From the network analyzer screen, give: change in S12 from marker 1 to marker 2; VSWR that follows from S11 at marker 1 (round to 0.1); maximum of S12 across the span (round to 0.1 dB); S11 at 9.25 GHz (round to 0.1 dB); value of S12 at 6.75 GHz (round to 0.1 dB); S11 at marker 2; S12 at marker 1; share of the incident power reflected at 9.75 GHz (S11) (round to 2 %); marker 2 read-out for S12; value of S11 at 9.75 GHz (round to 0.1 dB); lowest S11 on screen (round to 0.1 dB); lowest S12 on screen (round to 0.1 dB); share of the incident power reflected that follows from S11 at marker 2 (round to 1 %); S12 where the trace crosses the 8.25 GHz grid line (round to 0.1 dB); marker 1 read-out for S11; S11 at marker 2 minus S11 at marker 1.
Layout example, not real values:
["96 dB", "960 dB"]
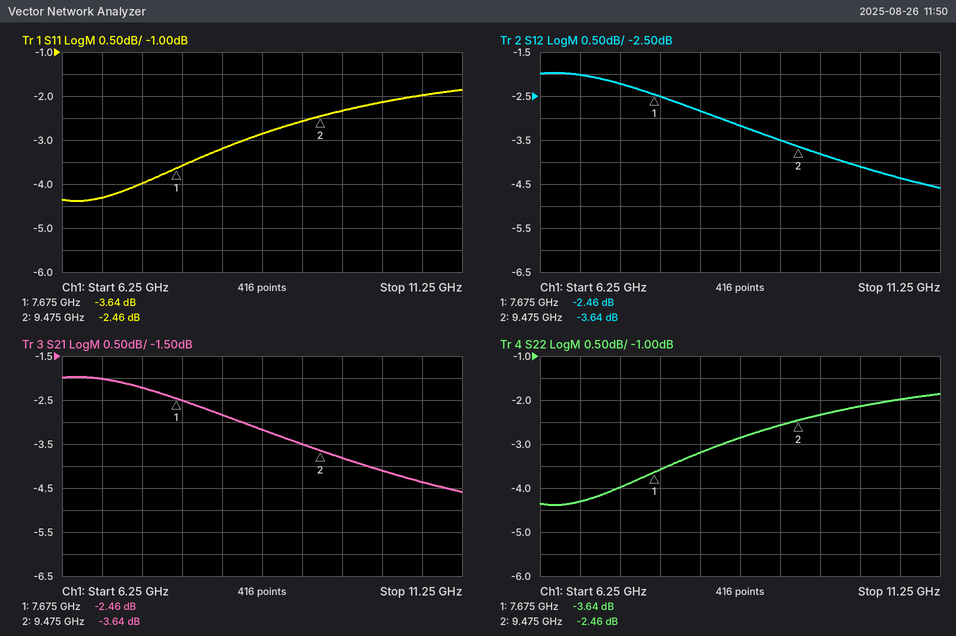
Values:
["-1.18 dB", "4.8", "-2.0 dB", "-2.6 dB", "-2.0 dB", "-2.46 dB", "-2.46 dB", "58 %", "-3.64 dB", "-2.3 dB", "-4.4 dB", "-4.6 dB", "57 %", "-2.8 dB", "-3.64 dB", "1.18 dB"]
